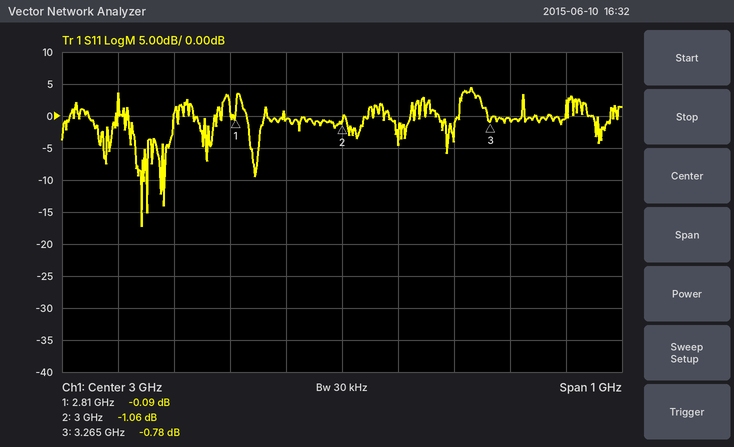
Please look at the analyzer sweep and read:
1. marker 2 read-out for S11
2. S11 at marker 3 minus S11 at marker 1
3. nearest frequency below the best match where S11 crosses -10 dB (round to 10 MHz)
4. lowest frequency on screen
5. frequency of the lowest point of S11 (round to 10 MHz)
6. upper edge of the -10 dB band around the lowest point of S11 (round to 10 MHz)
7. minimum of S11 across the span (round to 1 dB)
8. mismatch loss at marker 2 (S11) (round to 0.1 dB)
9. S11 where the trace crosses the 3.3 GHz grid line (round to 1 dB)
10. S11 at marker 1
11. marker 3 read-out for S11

-1.06 dB
-0.69 dB
2.64 GHz
2.5 GHz
2.64 GHz
2.64 GHz
-17 dB
6.6 dB
-1 dB
-0.09 dB
-0.78 dB
